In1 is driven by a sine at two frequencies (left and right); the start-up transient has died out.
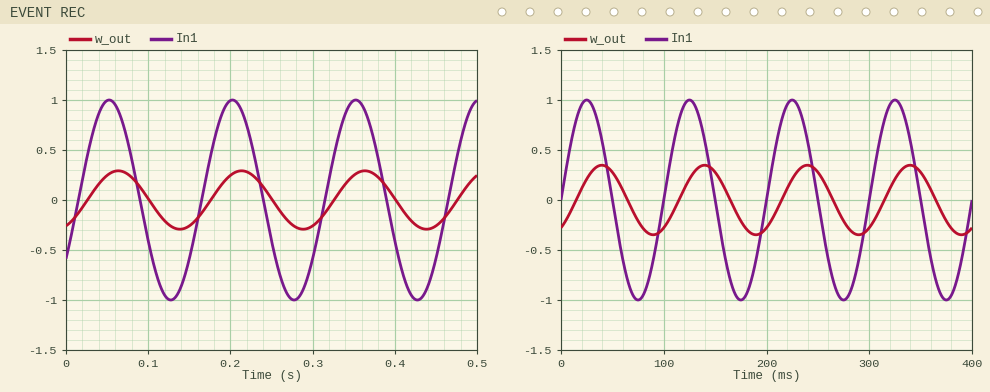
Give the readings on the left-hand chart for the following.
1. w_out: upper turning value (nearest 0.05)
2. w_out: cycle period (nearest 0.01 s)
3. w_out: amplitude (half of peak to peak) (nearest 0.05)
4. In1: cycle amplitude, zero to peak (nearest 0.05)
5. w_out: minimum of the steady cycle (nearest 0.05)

0.30
0.15 s
0.30
1.00
-0.30
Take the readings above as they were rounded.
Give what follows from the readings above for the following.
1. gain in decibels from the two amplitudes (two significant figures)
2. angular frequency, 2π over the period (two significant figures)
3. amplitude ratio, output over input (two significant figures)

-10 dB
42 rad/s
0.30
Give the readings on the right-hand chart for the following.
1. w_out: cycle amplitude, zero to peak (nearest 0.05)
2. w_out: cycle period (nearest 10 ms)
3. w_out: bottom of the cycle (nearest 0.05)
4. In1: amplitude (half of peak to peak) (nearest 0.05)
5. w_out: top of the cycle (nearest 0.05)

0.35
100 ms
-0.35
1.00
0.35
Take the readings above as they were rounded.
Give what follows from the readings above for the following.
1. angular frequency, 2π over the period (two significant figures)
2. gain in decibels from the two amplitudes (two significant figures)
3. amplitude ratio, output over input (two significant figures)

0.063 rad/ms
-9.1 dB
0.35
